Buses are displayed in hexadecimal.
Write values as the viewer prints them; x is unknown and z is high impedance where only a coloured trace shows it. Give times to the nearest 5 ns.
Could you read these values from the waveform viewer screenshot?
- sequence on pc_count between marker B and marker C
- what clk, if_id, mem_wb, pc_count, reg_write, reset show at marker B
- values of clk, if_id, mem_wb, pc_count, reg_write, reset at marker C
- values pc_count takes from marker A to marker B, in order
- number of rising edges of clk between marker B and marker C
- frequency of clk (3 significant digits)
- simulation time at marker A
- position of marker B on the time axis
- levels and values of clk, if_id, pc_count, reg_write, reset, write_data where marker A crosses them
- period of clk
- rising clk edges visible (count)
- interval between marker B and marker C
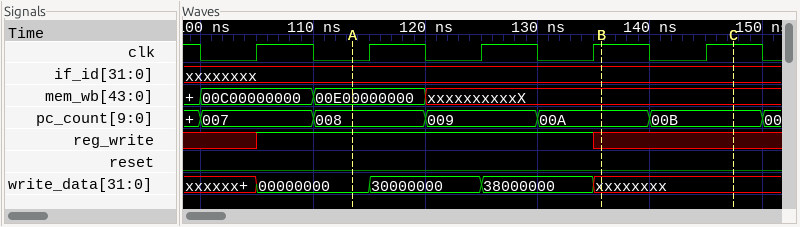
00A, 00B
clk=1, if_id=xxxxxxxx, mem_wb=xxxxxxxxxxX, pc_count=00A, reg_write=x, reset=0
clk=1, if_id=xxxxxxxx, mem_wb=xxxxxxxxxxX, pc_count=00B, reg_write=x, reset=0
008, 009, 00A
1
100 MHz
115 ns
135 ns
clk=0, if_id=xxxxxxxx, pc_count=008, reg_write=1, reset=0, write_data=00000000
10 ns
5
10 ns
